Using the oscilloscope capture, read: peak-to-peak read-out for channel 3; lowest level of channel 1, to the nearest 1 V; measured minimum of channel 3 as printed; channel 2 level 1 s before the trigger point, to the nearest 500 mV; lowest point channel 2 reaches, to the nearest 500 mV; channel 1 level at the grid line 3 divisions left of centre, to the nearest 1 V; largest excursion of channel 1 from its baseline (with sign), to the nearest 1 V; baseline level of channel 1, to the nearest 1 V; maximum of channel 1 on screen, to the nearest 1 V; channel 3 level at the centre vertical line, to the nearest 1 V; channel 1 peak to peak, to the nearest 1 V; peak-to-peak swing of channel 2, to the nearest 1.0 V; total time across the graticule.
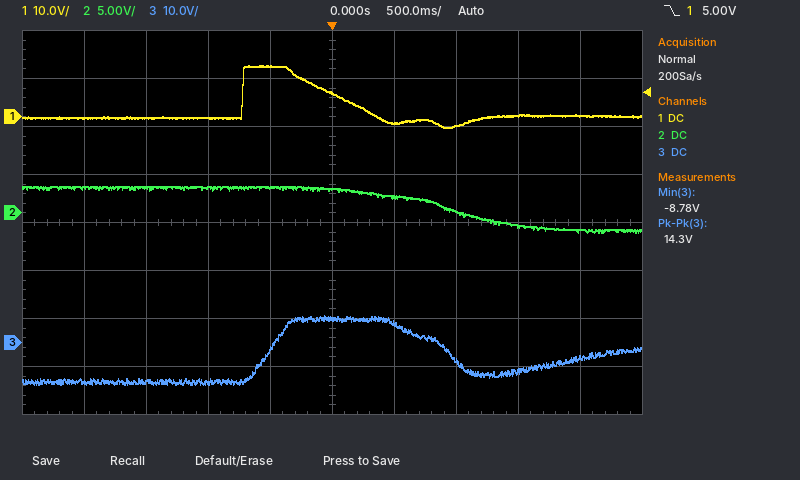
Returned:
14.3 V
-2 V
-8.78 V
2.5 V
-2.0 V
0 V
+11 V
0 V
11 V
5 V
13 V
5.0 V
5 s
